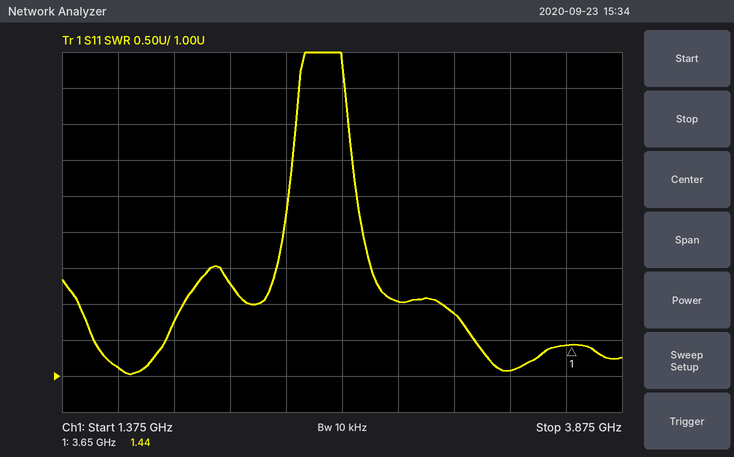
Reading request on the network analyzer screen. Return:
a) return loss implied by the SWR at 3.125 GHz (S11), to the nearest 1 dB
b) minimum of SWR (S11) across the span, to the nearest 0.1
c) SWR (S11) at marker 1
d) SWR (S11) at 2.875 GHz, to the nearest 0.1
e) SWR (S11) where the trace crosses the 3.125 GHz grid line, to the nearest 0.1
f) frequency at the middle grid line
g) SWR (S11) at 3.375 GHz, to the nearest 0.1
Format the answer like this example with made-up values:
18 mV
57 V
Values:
10 dB
1.0
1.44
2.0
1.9
2.625 GHz
1.1
